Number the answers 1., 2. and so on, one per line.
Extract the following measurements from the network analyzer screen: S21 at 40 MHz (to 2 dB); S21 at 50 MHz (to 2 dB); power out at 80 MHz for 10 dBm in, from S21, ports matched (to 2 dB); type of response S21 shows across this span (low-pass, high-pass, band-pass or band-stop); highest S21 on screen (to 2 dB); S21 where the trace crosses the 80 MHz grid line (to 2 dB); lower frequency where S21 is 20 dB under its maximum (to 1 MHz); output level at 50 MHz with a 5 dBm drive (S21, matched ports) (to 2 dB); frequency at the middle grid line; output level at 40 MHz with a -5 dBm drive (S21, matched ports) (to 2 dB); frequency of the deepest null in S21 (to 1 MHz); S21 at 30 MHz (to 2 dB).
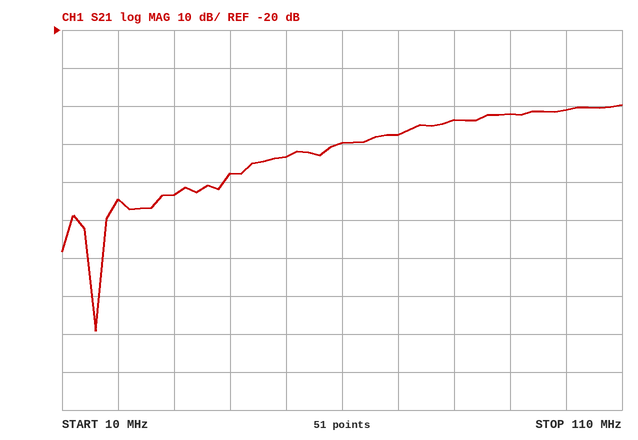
1. -58 dB
2. -54 dB
3. -34 dBm
4. high-pass
5. -40 dB
6. -44 dB
7. 39 MHz
8. -48 dBm
9. 60 MHz
10. -62 dBm
11. 16 MHz
12. -64 dB
